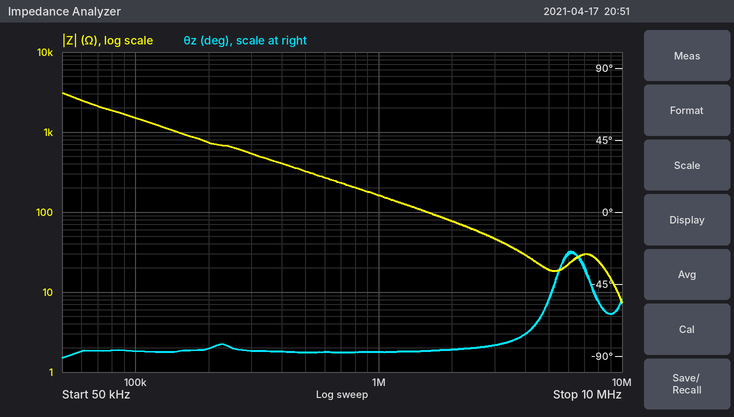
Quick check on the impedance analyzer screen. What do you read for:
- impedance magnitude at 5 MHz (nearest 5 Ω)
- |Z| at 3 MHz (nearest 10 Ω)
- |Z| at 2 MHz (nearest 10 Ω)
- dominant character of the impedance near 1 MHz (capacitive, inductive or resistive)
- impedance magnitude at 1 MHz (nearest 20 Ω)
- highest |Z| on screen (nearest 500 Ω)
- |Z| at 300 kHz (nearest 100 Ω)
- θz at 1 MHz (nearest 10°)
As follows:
20 Ω
50 Ω
80 Ω
capacitive
160 Ω
3.0 kΩ
500 Ω
-90°
